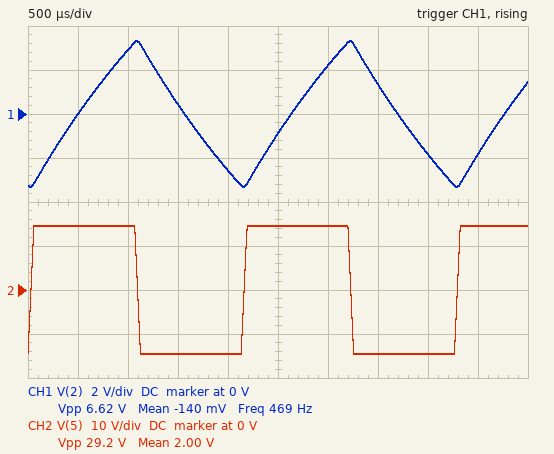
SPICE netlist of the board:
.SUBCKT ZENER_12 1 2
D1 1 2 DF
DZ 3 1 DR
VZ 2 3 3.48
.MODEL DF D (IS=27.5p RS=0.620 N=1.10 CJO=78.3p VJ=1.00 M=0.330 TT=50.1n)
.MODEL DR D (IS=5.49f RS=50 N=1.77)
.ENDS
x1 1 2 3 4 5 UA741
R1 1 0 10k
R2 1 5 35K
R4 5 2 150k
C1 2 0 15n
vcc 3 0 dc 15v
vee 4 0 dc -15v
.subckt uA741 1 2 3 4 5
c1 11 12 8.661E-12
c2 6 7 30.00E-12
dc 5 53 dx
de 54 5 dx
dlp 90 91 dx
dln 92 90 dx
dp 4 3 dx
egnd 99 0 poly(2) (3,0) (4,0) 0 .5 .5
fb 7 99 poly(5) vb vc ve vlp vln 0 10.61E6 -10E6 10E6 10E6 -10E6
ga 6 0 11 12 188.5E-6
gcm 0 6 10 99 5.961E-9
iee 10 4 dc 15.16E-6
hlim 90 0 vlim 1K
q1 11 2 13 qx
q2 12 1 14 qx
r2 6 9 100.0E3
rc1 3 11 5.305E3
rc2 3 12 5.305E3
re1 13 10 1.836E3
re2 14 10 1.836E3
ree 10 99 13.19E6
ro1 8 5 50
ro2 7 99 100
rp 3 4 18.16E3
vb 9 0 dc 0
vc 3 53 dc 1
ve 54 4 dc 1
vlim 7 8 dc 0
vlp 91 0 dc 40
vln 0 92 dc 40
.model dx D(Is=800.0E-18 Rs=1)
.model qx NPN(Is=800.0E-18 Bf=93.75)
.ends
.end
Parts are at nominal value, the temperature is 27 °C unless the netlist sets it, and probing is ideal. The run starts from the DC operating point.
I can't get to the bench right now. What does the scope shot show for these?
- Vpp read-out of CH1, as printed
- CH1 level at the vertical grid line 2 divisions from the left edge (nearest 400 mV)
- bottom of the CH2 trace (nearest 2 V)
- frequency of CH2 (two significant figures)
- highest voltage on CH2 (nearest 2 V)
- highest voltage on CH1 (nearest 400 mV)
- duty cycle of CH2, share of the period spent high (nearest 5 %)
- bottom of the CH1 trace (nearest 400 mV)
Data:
6.62 V
2.8 V
-14 V
470 Hz
14 V
3.2 V
50 %
-3.2 V
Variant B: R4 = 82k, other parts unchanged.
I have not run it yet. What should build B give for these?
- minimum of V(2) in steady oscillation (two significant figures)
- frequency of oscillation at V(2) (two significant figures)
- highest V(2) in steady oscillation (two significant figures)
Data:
-3.4 V
820 Hz
3.4 V
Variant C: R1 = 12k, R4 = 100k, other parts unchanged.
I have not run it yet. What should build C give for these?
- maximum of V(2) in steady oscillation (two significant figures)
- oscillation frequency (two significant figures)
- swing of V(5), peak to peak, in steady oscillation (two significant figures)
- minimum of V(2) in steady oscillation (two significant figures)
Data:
3.8 V
600 Hz
29 V
-3.8 V
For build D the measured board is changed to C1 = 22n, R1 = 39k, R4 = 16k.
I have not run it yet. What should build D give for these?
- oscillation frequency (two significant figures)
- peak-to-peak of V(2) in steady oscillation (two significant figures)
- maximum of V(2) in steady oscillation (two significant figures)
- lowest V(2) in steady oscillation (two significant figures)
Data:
1.1 kHz
16 V
7.9 V
-7.9 V
